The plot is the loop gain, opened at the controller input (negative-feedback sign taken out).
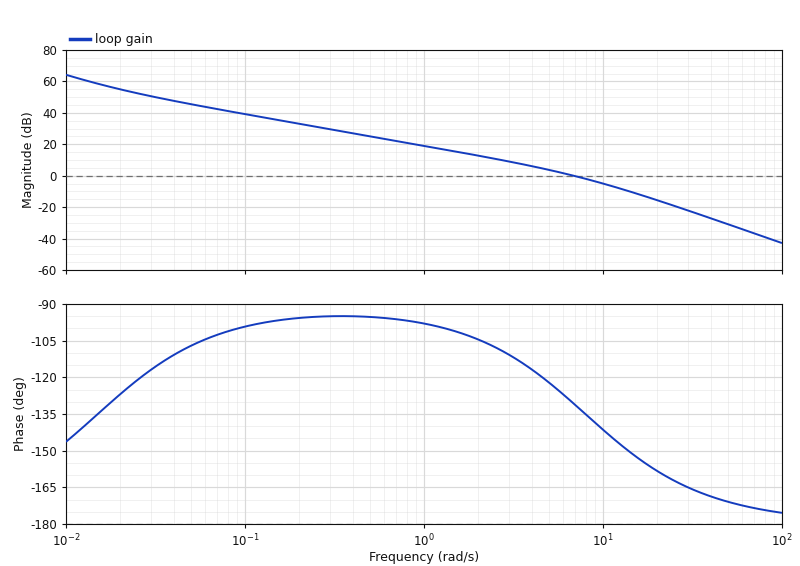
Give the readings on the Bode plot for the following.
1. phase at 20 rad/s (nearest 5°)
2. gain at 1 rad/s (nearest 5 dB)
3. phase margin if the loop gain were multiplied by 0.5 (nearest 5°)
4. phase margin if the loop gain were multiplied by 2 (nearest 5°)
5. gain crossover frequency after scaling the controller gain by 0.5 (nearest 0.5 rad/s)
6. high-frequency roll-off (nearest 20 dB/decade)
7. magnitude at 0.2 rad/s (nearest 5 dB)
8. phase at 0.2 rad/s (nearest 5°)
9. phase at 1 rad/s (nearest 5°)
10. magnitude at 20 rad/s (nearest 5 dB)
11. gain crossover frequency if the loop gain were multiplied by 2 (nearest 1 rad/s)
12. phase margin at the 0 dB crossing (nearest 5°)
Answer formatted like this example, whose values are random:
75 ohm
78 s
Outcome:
-160°
20 dB
65°
35°
4.0 rad/s
-40 dB/decade
35 dB
-95°
-100°
-15 dB
11 rad/s
50°
